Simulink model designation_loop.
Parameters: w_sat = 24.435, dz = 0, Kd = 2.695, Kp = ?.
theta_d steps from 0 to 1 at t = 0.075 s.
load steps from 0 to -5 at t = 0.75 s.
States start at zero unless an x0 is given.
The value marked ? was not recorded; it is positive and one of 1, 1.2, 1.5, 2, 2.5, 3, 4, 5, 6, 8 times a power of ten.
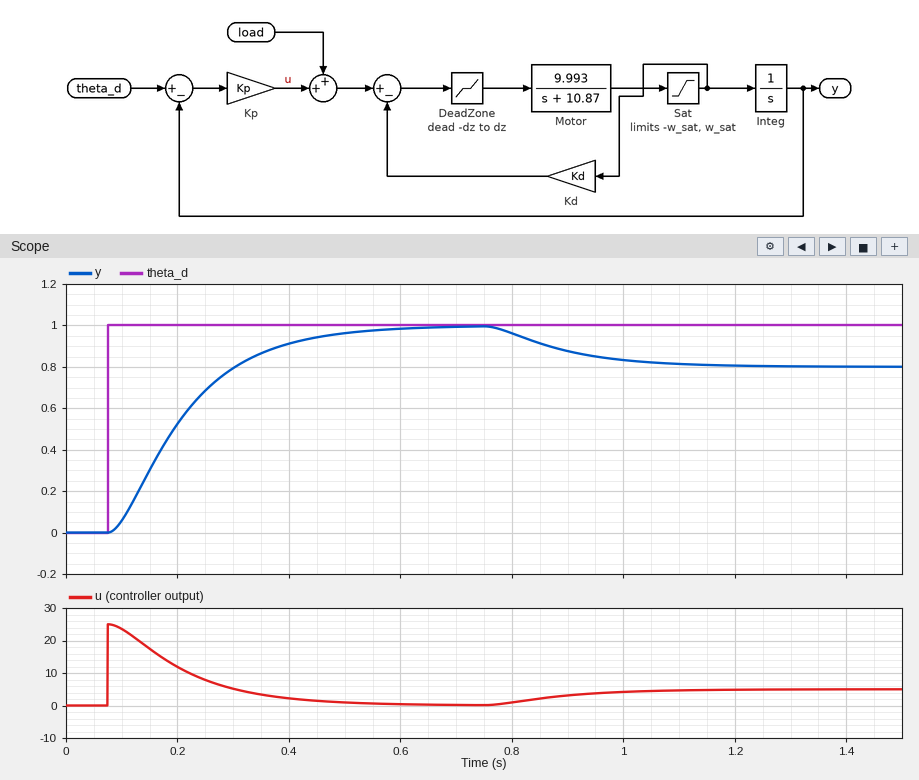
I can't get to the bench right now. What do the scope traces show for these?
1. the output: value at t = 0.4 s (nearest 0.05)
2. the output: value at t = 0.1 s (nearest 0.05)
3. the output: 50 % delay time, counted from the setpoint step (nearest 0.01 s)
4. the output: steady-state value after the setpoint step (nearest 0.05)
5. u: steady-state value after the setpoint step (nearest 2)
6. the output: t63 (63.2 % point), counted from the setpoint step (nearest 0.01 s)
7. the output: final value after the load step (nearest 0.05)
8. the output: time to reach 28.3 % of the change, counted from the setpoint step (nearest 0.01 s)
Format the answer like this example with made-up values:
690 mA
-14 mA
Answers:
0.90
0.05
0.12 s
1.00
0
0.16 s
0.80
0.07 s
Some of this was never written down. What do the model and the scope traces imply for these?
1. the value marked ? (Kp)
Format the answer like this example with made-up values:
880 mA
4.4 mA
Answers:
25
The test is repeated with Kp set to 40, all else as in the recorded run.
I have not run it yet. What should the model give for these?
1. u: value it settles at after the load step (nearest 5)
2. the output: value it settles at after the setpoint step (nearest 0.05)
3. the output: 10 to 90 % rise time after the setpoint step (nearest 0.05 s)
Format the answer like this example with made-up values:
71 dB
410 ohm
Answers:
5
1.00
0.15 s
